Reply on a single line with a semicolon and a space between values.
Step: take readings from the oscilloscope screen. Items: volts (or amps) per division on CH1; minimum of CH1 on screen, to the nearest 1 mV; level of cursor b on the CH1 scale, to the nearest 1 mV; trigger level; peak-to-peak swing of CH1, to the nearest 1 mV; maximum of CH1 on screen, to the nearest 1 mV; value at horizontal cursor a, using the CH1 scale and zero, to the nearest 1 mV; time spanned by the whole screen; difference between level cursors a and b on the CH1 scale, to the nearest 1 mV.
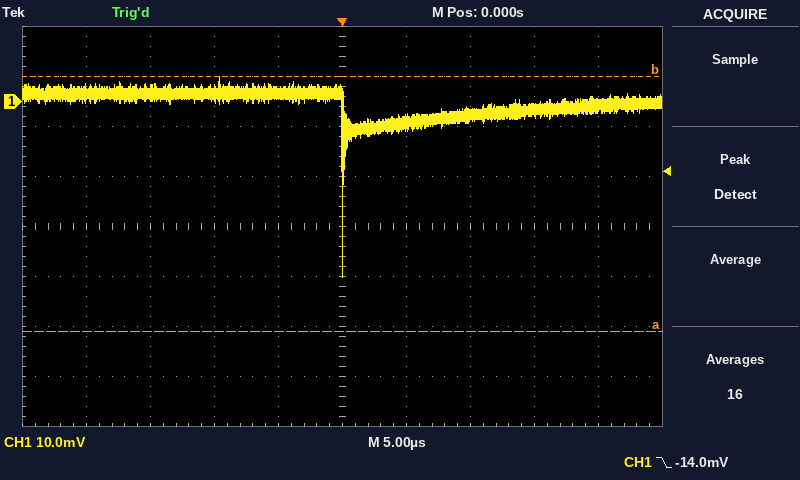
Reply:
10 mV; -35 mV; 5 mV; -14.0 mV; 40 mV; 5 mV; -46 mV; 50 µs; 51 mV
